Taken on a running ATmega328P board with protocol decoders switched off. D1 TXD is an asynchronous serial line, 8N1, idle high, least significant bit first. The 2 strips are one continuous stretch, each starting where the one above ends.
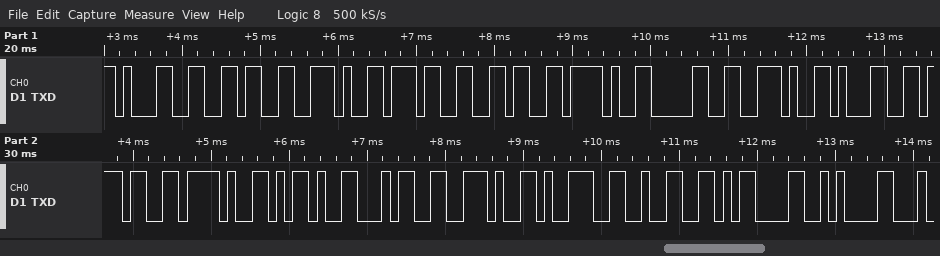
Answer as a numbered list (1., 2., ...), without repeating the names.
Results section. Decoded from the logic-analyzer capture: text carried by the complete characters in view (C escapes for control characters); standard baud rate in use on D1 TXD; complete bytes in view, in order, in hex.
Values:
1. "16.76/0.17/-4.92\r\n"
2. 9600 baud
3. 0x31 0x36 0x2E 0x37 0x36 0x2F 0x30 0x2E 0x31 0x37 0x2F 0x2D 0x34 0x2E 0x39 0x32 0x0D 0x0A
